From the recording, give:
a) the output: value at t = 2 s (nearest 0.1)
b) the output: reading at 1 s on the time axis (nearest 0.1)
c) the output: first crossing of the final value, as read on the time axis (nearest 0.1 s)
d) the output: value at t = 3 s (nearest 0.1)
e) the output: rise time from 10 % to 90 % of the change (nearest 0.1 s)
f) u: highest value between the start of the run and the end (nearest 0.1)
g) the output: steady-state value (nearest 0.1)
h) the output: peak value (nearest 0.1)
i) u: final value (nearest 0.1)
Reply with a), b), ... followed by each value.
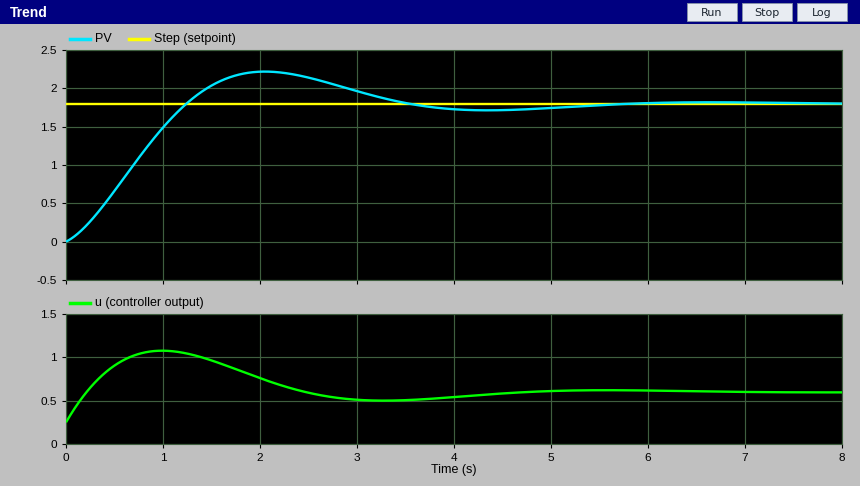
a) 2.2
b) 1.5
c) 1.2 s
d) 2.0
e) 0.9 s
f) 1.1
g) 1.8
h) 2.2
i) 0.6
